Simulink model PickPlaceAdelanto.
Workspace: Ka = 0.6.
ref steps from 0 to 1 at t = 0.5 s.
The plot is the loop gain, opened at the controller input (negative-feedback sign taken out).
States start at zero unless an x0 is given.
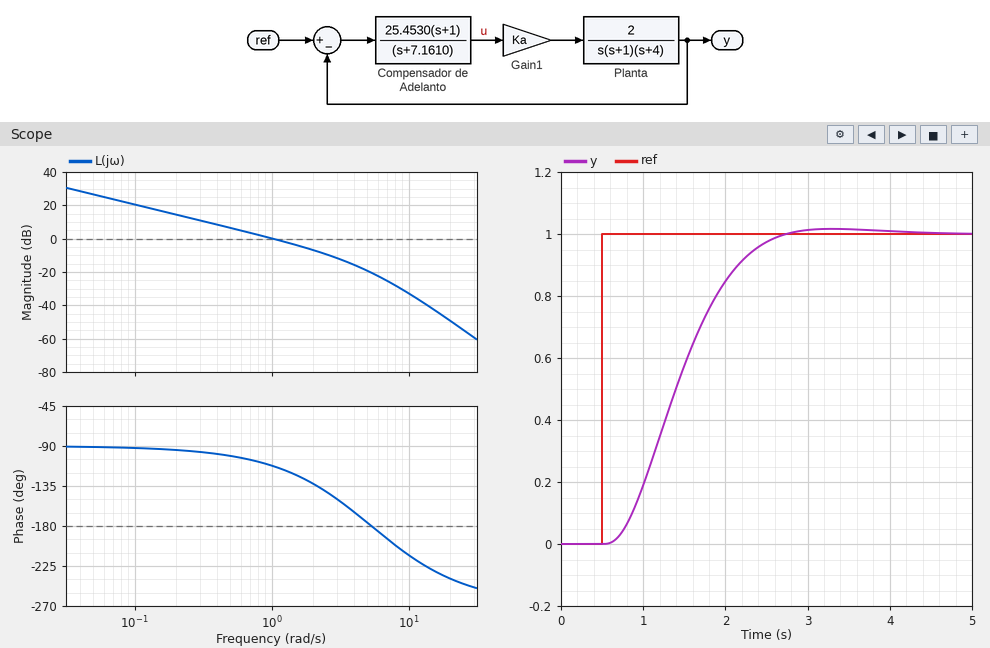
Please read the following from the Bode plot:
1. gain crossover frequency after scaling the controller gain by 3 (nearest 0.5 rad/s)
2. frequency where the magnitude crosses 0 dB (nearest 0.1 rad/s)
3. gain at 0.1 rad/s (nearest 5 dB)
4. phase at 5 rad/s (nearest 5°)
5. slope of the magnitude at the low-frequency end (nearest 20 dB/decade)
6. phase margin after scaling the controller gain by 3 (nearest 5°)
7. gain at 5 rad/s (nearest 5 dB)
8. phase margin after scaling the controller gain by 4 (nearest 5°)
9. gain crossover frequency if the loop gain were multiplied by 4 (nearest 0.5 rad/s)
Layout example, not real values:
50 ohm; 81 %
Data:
2.5 rad/s; 1.0 rad/s; 20 dB; -175°; -20 dB/decade; 40°; -20 dB; 30°; 3.0 rad/s
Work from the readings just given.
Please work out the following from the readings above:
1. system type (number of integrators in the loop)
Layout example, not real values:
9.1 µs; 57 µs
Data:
1
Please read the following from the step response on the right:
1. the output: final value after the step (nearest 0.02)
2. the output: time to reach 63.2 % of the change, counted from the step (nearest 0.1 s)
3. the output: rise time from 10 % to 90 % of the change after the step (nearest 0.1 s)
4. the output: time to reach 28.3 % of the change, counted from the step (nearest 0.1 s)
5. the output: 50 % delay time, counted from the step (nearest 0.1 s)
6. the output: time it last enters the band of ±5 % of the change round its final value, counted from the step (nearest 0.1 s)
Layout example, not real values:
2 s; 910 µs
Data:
1.00; 1.1 s; 1.3 s; 0.6 s; 0.9 s; 1.9 s
